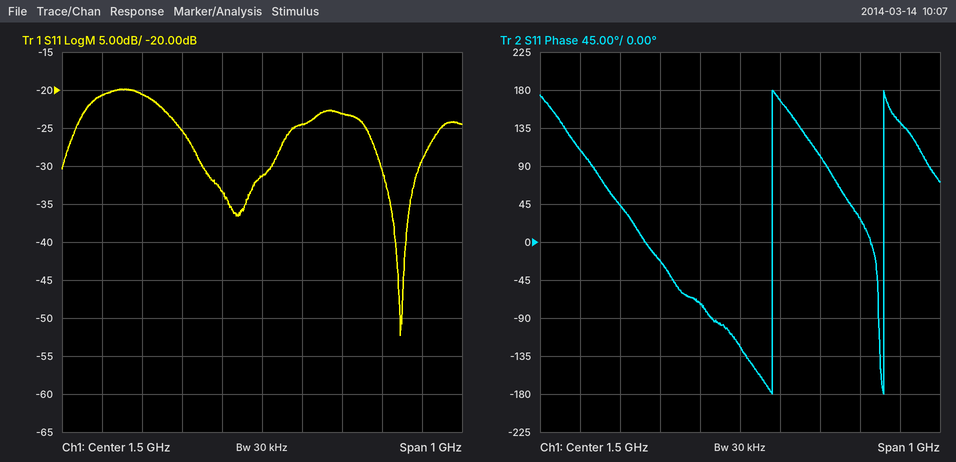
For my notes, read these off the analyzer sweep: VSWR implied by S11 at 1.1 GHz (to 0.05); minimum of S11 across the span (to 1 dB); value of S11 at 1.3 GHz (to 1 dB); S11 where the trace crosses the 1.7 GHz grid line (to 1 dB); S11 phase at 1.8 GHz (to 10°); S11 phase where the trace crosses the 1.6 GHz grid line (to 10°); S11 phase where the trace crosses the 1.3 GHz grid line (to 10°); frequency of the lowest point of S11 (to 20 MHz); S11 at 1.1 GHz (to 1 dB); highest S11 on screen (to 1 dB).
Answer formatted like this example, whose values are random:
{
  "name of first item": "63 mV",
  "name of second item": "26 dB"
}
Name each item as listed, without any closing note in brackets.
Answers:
{
  "VSWR implied by S11 at 1.1 GHz": "1.20",
  "minimum of S11 across the span": "-52 dB",
  "value of S11 at 1.3 GHz": "-25 dB",
  "S11 where the trace crosses the 1.7 GHz grid line": "-23 dB",
  "S11 phase at 1.8 GHz": "30°",
  "S11 phase where the trace crosses the 1.6 GHz grid line": "170°",
  "S11 phase where the trace crosses the 1.3 GHz grid line": "-20°",
  "frequency of the lowest point of S11": "1.84 GHz",
  "S11 at 1.1 GHz": "-21 dB",
  "highest S11 on screen": "-20 dB"
}
